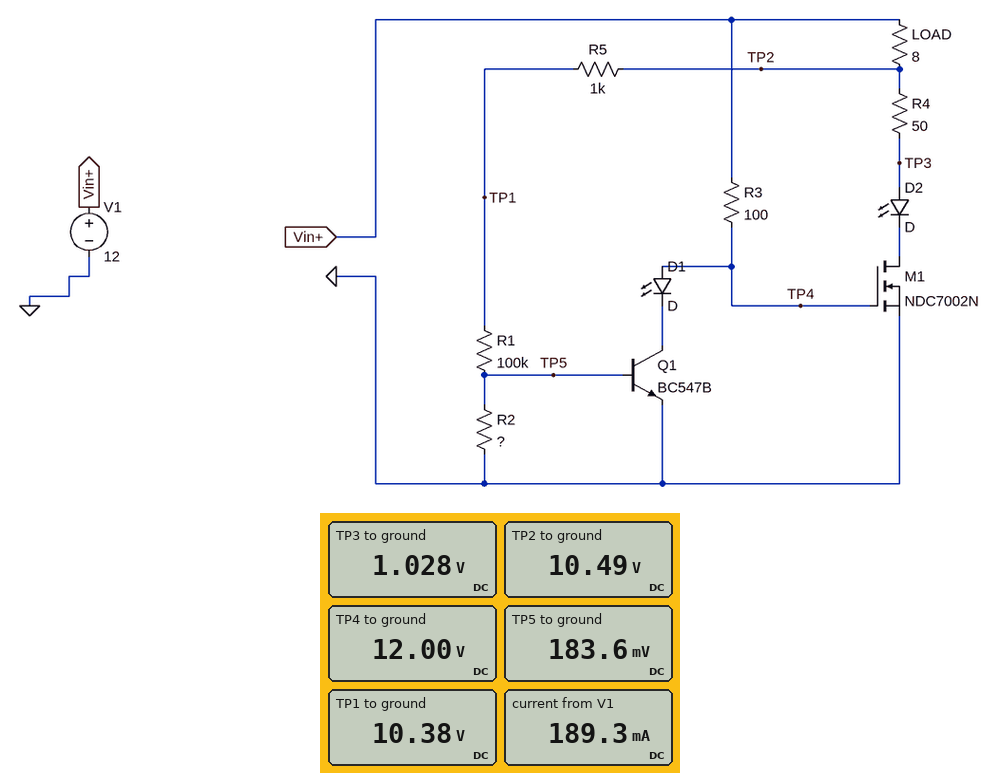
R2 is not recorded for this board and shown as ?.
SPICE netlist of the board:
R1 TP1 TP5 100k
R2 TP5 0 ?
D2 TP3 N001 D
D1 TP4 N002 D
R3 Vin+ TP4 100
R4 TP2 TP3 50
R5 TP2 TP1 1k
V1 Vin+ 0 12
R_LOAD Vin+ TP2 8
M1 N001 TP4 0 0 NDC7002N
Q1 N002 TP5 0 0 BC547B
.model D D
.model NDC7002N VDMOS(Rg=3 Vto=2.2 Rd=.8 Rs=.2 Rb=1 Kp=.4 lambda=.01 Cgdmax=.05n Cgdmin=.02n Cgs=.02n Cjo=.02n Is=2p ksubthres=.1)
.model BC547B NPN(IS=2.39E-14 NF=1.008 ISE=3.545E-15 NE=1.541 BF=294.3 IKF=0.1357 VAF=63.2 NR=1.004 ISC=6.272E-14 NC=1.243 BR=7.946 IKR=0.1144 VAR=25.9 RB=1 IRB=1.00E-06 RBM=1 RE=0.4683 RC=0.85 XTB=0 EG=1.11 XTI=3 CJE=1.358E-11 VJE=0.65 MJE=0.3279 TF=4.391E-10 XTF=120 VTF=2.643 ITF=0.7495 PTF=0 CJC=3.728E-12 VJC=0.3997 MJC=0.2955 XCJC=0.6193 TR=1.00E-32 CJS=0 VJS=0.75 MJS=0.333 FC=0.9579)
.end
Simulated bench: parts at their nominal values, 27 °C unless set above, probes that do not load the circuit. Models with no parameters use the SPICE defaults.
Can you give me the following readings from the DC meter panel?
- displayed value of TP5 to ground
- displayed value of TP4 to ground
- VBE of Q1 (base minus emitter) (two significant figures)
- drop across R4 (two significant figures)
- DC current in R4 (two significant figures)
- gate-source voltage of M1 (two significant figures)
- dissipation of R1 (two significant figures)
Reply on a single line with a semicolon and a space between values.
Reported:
183.6 mV; 12.00 V; 180 mV; 9.5 V; 190 mA; 12 V; 1.0 mW
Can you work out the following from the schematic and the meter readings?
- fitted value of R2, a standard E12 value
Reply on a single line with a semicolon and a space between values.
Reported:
1.8 kΩ
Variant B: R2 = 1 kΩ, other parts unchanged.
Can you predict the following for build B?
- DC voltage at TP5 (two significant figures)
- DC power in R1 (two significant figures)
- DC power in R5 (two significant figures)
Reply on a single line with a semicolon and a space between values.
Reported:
100 mV; 1.1 mW; 11 µW
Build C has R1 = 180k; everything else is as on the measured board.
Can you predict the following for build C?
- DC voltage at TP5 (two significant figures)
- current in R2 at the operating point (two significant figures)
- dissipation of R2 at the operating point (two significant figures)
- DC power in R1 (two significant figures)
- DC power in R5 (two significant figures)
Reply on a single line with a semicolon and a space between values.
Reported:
100 mV; 57 µA; 5.9 µW; 590 µW; 3.3 µW
